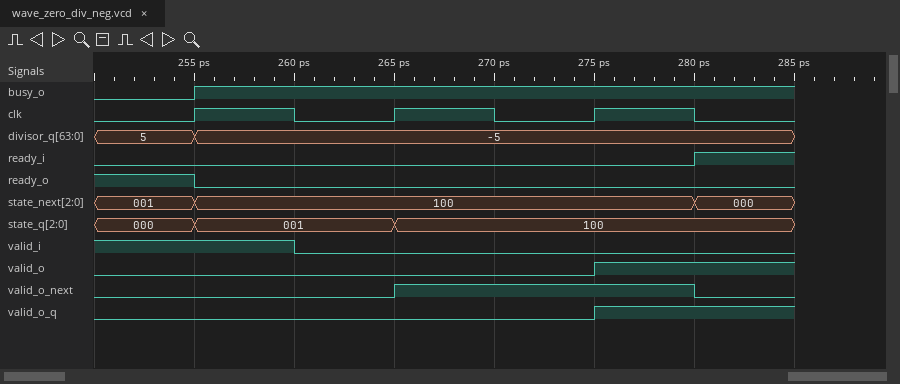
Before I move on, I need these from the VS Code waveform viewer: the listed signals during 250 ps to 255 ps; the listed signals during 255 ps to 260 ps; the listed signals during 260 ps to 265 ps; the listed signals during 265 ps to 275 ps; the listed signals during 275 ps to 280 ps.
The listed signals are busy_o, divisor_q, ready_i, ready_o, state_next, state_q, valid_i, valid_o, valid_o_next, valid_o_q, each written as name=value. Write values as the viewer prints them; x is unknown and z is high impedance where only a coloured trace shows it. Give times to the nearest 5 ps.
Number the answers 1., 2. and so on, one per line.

1. busy_o=0, divisor_q=5, ready_i=0, ready_o=1, state_next=001, state_q=000, valid_i=1, valid_o=0, valid_o_next=0, valid_o_q=0
2. busy_o=1, divisor_q=-5, ready_i=0, ready_o=0, state_next=100, state_q=001, valid_i=1, valid_o=0, valid_o_next=0, valid_o_q=0
3. busy_o=1, divisor_q=-5, ready_i=0, ready_o=0, state_next=100, state_q=001, valid_i=0, valid_o=0, valid_o_next=0, valid_o_q=0
4. busy_o=1, divisor_q=-5, ready_i=0, ready_o=0, state_next=100, state_q=100, valid_i=0, valid_o=0, valid_o_next=1, valid_o_q=0
5. busy_o=1, divisor_q=-5, ready_i=0, ready_o=0, state_next=100, state_q=100, valid_i=0, valid_o=1, valid_o_next=1, valid_o_q=1
